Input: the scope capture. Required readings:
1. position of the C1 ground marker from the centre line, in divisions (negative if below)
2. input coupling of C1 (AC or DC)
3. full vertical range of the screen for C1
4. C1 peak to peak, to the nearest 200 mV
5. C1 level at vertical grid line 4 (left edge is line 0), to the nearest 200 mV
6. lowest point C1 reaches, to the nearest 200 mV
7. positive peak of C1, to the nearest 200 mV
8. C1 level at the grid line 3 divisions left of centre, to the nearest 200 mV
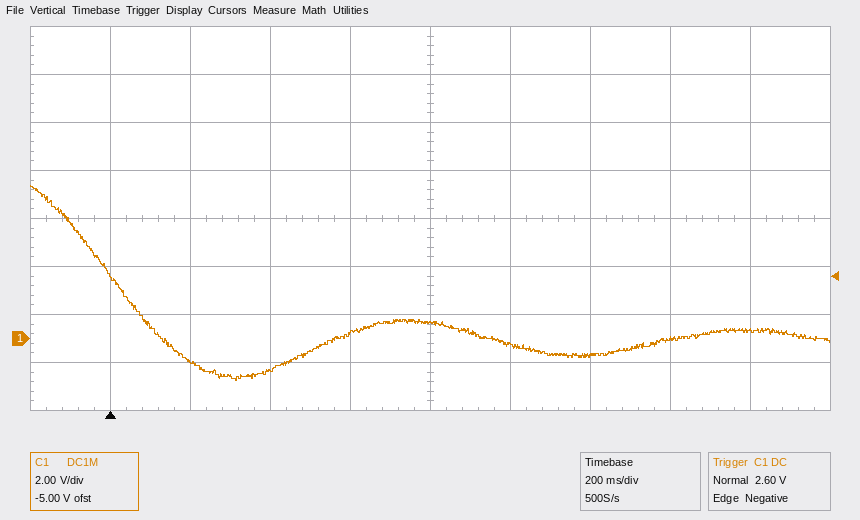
-2.5 div
DC
16 V
8.2 V
200 mV
-1.8 V
6.4 V
-1.0 V
